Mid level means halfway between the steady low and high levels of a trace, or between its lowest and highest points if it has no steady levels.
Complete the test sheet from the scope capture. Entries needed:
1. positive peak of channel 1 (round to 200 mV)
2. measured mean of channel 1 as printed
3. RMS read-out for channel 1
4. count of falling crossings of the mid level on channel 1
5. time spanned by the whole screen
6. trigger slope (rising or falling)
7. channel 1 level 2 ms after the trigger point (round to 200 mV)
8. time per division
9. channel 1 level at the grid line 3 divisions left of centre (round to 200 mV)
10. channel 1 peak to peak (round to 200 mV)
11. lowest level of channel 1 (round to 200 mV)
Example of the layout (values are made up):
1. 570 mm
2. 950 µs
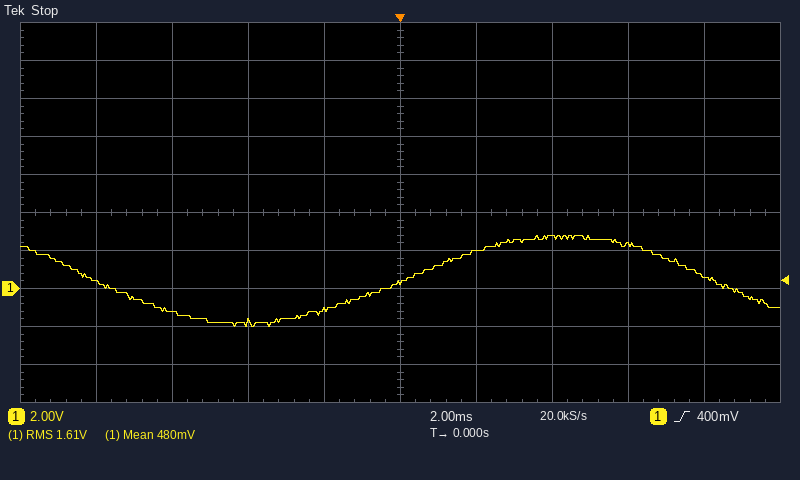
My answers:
1. 2.8 V
2. 480 mV
3. 1.61 V
4. 2
5. 20 ms
6. rising
7. 2.0 V
8. 2 ms
9. -1.2 V
10. 4.8 V
11. -2.0 V
